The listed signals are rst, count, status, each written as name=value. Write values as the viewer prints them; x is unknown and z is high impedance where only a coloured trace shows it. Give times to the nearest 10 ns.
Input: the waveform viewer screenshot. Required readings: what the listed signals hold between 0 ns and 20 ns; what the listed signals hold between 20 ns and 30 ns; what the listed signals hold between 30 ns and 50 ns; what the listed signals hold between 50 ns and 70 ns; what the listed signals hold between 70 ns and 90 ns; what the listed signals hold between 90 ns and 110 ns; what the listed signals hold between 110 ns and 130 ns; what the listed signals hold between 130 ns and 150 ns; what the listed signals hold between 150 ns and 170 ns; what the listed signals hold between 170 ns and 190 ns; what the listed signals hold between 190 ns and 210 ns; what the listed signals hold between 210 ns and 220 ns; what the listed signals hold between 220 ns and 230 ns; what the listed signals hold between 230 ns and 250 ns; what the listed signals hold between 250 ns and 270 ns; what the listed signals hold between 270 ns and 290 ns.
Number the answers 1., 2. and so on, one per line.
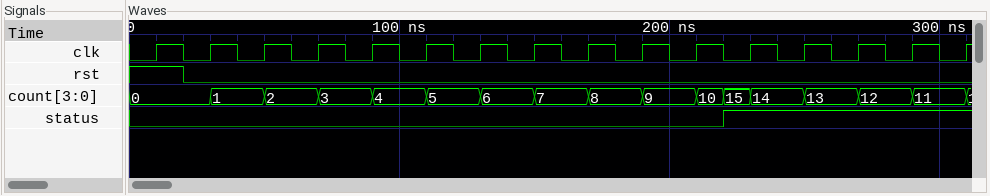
1. rst=1, count=0, status=0
2. rst=0, count=0, status=0
3. rst=0, count=1, status=0
4. rst=0, count=2, status=0
5. rst=0, count=3, status=0
6. rst=0, count=4, status=0
7. rst=0, count=5, status=0
8. rst=0, count=6, status=0
9. rst=0, count=7, status=0
10. rst=0, count=8, status=0
11. rst=0, count=9, status=0
12. rst=0, count=10, status=0
13. rst=0, count=15, status=1
14. rst=0, count=14, status=1
15. rst=0, count=13, status=1
16. rst=0, count=12, status=1
